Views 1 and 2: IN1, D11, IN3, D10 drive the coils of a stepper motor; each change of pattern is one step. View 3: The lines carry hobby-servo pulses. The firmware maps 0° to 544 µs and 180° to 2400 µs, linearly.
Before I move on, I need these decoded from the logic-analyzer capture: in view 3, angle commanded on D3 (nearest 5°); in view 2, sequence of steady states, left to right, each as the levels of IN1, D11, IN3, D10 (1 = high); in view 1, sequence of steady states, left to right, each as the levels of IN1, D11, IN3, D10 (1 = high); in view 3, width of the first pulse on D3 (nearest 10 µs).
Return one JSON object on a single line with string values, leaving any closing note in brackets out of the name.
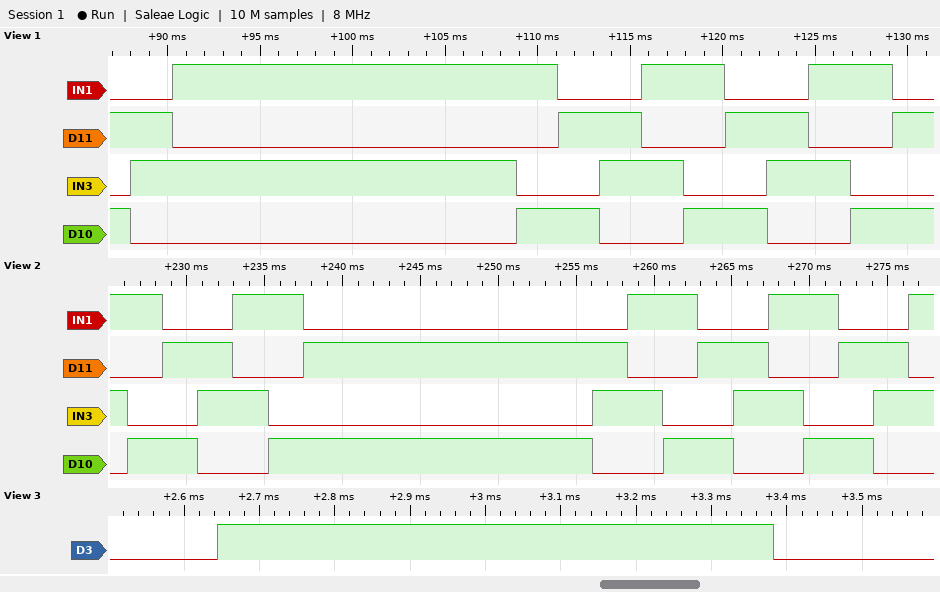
{"in view 3, angle commanded on D3": "20°", "in view 2, sequence of steady states, left to right, each as the levels of IN1, D11, IN3, D10": "1010 1001 0101 0110 1010 1001 0101 0110 1010 1001 0101 0110 1010 1001 0101 0110 1010", "in view 1, sequence of steady states, left to right, each as the levels of IN1, D11, IN3, D10": "0101 0110 1010 1001 0101 0110 1010 1001 0101 0110 1010 1001 0101", "in view 3, width of the first pulse on D3": "740 µs"}
